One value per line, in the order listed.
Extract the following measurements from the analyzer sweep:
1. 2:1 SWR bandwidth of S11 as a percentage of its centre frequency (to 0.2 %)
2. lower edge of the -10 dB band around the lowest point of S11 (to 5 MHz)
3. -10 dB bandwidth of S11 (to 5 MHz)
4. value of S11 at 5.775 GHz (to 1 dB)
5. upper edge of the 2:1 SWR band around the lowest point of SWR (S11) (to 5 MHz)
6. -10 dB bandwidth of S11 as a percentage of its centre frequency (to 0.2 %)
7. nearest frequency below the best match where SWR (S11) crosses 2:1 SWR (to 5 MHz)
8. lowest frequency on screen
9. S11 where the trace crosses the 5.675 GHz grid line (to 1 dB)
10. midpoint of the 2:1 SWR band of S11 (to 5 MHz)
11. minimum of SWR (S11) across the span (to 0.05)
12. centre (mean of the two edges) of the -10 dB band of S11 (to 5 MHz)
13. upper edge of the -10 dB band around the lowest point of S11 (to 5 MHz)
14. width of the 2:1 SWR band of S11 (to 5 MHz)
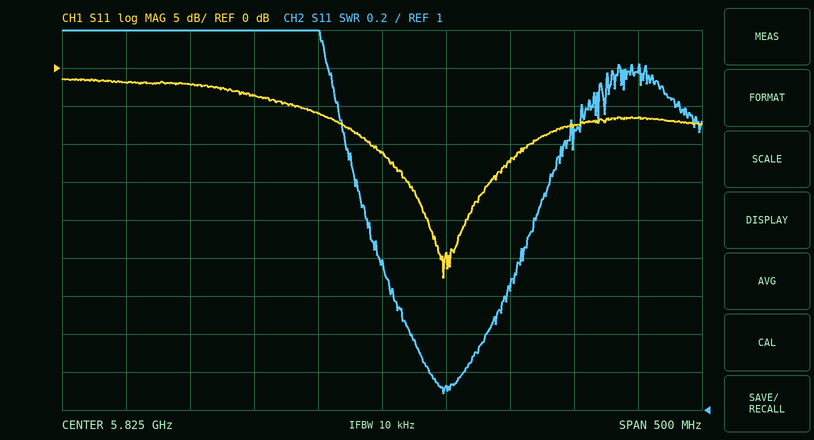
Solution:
2.2 %
5.815 GHz
125 MHz
-6 dB
5.945 GHz
2.2 %
5.815 GHz
5.575 GHz
-2 dB
5.880 GHz
1.10
5.880 GHz
5.940 GHz
130 MHz
